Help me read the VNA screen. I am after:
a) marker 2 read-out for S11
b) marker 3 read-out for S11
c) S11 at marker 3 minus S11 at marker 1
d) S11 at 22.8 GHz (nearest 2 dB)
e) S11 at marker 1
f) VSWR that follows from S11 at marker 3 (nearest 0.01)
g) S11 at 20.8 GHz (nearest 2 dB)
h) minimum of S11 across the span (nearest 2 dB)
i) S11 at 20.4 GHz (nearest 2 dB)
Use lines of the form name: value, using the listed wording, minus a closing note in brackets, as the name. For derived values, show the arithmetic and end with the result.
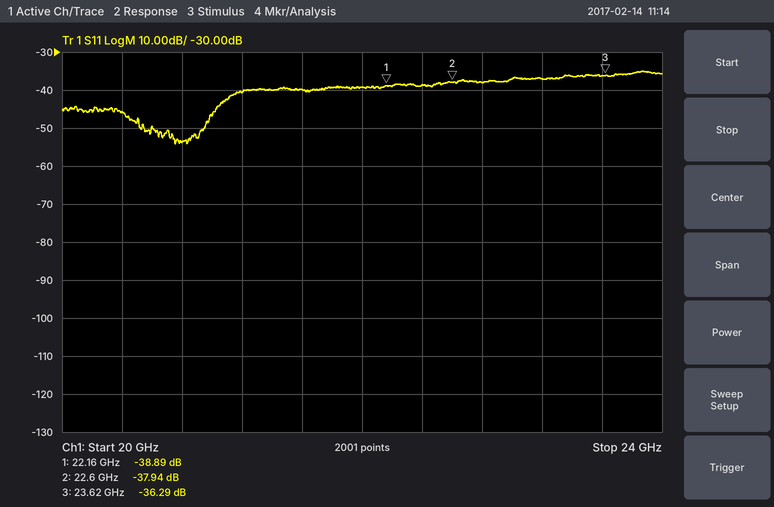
marker 2 read-out for S11: -37.94 dB
marker 3 read-out for S11: -36.29 dB
S11 at marker 3 minus S11 at marker 1: -36.29 − (-38.89) = 2.60 dB
S11 at 22.8 GHz: -38 dB
S11 at marker 1: -38.89 dB
VSWR that follows from S11 at marker 3: (1 + 0.0153)/(1 − 0.0153) ≈ 1.03
S11 at 20.8 GHz: -54 dB
minimum of S11 across the span: -54 dB
S11 at 20.4 GHz: -46 dB
